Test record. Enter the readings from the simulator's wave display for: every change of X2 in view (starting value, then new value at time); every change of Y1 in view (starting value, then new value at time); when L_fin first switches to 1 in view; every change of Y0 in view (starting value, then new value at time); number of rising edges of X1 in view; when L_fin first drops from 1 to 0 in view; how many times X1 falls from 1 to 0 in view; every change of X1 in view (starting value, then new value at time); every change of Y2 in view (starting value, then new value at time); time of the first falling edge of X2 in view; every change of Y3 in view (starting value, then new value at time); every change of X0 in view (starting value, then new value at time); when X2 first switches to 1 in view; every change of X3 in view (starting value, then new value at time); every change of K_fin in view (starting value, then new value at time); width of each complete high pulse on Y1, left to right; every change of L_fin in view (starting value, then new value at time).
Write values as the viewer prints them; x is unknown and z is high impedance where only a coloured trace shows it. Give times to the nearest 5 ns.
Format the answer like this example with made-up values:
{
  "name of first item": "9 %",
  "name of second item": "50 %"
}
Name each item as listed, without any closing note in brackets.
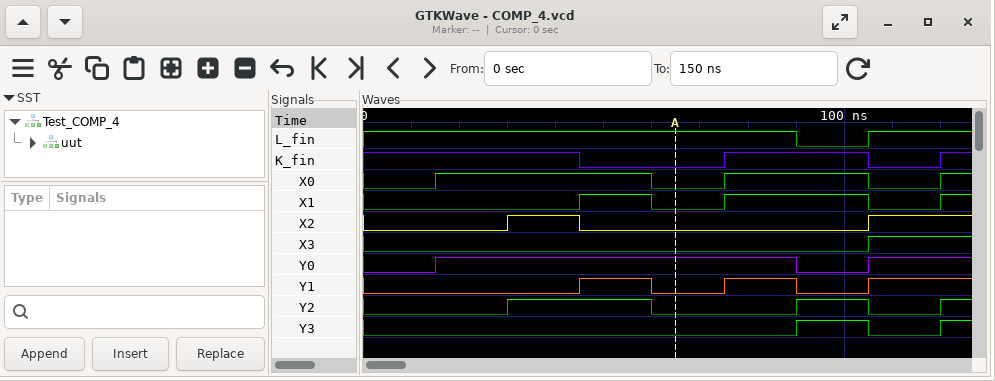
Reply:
{
  "every change of X2 in view": "0, 1 at 30 ns, 0 at 45 ns, 1 at 105 ns",
  "every change of Y1 in view": "0, 1 at 45 ns, 0 at 60 ns, 1 at 75 ns, 0 at 90 ns, 1 at 105 ns",
  "when L_fin first switches to 1 in view": "105 ns",
  "every change of Y0 in view": "0, 1 at 15 ns, 0 at 90 ns, 1 at 105 ns",
  "number of rising edges of X1 in view": "3",
  "when L_fin first drops from 1 to 0 in view": "90 ns",
  "how many times X1 falls from 1 to 0 in view": "2",
  "every change of X1 in view": "0, 1 at 45 ns, 0 at 60 ns, 1 at 75 ns, 0 at 105 ns, 1 at 120 ns",
  "every change of Y2 in view": "0, 1 at 30 ns, 0 at 60 ns, 1 at 90 ns, 0 at 105 ns, 1 at 120 ns",
  "time of the first falling edge of X2 in view": "45 ns",
  "every change of Y3 in view": "0, 1 at 90 ns, 0 at 105 ns, 1 at 120 ns",
  "every change of X0 in view": "0, 1 at 15 ns, 0 at 60 ns, 1 at 75 ns, 0 at 105 ns, 1 at 120 ns",
  "when X2 first switches to 1 in view": "30 ns",
  "every change of X3 in view": "0, 1 at 105 ns",
  "every change of K_fin in view": "1, 0 at 45 ns, 1 at 75 ns, 0 at 105 ns, 1 at 120 ns",
  "width of each complete high pulse on Y1, left to right": "15 ns, 15 ns",
  "every change of L_fin in view": "1, 0 at 90 ns, 1 at 105 ns"
}
